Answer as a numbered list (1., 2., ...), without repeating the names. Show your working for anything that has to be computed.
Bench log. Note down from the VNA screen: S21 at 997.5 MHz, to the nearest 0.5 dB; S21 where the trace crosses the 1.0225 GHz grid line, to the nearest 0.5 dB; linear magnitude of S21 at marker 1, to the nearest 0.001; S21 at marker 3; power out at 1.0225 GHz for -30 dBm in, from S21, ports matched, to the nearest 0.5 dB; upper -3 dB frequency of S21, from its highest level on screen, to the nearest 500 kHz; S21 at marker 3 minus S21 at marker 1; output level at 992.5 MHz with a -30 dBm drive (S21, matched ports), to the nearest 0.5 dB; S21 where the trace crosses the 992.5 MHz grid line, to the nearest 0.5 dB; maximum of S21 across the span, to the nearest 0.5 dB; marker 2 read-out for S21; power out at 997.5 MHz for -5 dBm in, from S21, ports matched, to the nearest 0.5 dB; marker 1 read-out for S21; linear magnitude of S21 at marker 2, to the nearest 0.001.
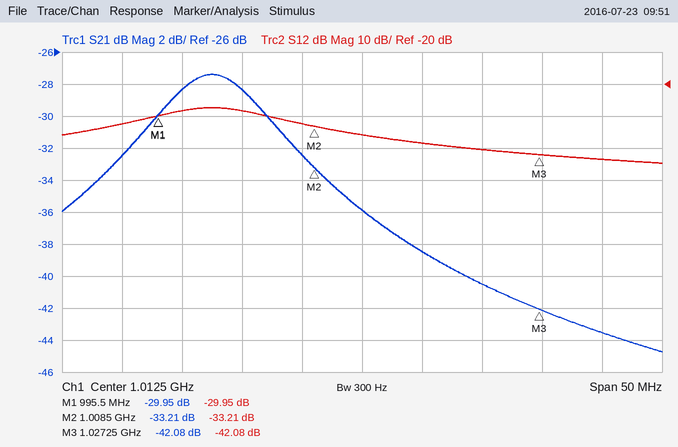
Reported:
1. -28.5 dB
2. -40.5 dB
3. 10^(-29.95/20) ≈ 0.032
4. -42.08 dB
5. -30 dBm + (-40.5 dB) = -70.5 dBm
6. 1.0050 GHz
7. -42.08 − (-29.95) = -12.13 dB
8. -30 dBm + (-32.5 dB) = -62.5 dBm
9. -32.5 dB
10. -27.5 dB
11. -33.21 dB
12. -5 dBm + (-28.5 dB) = -33.5 dBm
13. -29.95 dB
14. 10^(-33.21/20) ≈ 0.022
